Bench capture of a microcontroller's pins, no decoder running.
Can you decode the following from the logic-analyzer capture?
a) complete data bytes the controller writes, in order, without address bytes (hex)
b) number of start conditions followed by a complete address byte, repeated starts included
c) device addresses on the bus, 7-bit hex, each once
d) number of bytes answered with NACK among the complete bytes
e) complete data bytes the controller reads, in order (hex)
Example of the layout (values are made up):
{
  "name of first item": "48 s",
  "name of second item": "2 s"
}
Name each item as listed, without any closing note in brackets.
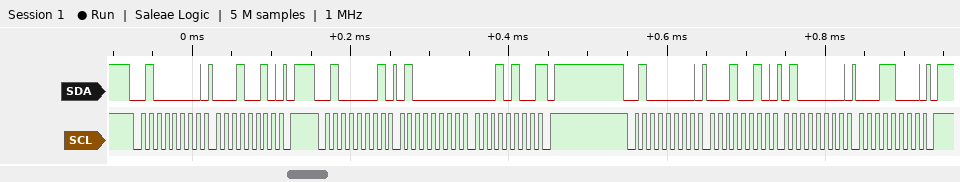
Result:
{
  "complete data bytes the controller writes, in order, without address bytes": "12 12 40 18",
  "number of start conditions followed by a complete address byte, repeated starts included": "3",
  "device addresses on the bus, 7-bit hex, each once": "0x20",
  "number of bytes answered with NACK among the complete bytes": "1",
  "complete data bytes the controller reads, in order": "40 14"
}
